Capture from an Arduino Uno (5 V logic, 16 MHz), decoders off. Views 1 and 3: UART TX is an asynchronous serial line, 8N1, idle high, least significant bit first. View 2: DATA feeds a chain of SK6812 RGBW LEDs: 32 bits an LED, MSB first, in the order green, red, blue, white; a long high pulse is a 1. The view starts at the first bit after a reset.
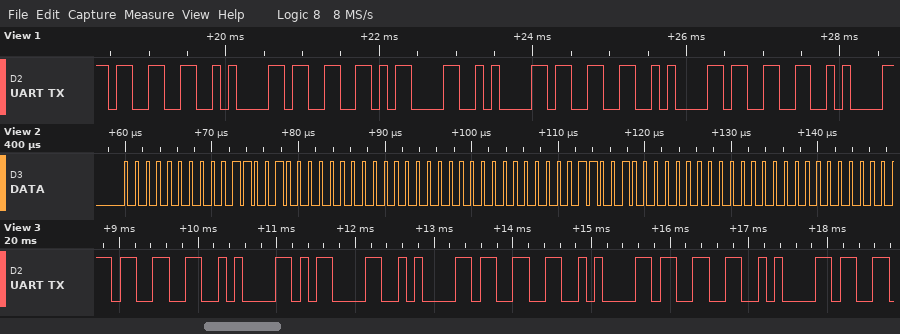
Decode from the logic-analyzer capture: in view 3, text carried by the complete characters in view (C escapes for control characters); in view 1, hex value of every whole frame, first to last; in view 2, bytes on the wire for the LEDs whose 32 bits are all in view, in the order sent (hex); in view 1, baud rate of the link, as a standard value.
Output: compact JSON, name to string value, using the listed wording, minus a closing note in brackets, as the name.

{"in view 3, text carried by the complete characters in view": "\"3\\n\\r\\n3\\n3\\n\"", "in view 1, hex value of every whole frame, first to last": "33 0A 33 0D 0A 33 0A 33 0A", "in view 2, bytes on the wire for the LEDs whose 32 bits are all in view, in the order sent": "00 32 00 00 00 32 00 00", "in view 1, baud rate of the link, as a standard value": "9600 baud"}
